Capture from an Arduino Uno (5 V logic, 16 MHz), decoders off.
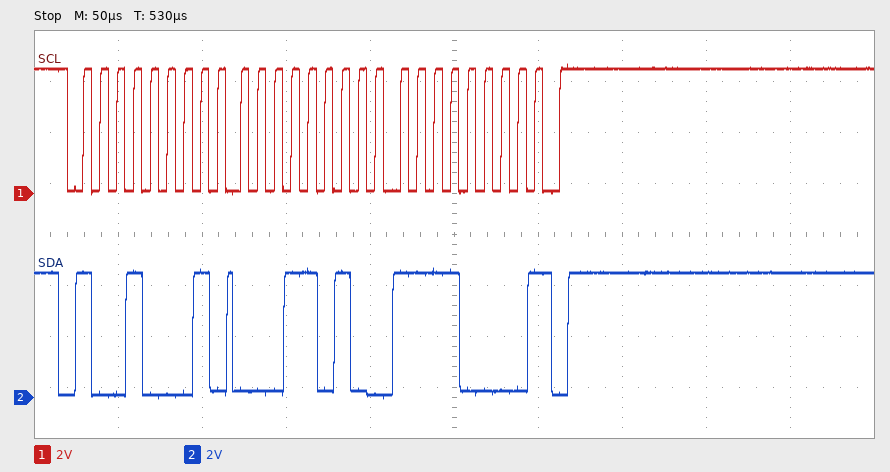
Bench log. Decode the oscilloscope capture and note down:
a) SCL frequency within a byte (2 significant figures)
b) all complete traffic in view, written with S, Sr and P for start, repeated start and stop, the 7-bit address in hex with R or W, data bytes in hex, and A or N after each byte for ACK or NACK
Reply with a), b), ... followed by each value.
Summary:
a) 100 kHz
b) S 48R A 1A A F0 N P
